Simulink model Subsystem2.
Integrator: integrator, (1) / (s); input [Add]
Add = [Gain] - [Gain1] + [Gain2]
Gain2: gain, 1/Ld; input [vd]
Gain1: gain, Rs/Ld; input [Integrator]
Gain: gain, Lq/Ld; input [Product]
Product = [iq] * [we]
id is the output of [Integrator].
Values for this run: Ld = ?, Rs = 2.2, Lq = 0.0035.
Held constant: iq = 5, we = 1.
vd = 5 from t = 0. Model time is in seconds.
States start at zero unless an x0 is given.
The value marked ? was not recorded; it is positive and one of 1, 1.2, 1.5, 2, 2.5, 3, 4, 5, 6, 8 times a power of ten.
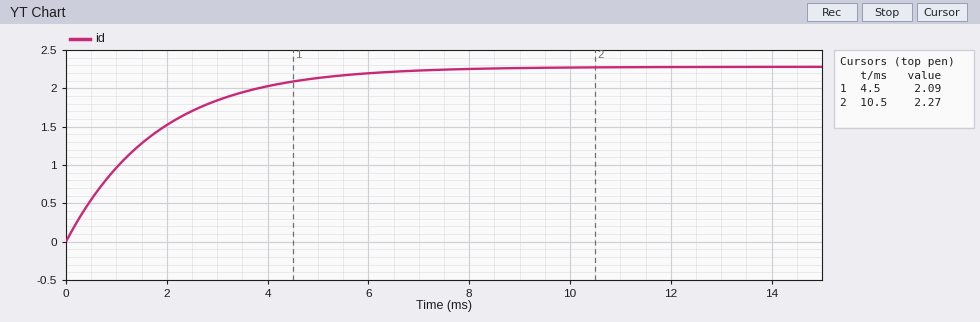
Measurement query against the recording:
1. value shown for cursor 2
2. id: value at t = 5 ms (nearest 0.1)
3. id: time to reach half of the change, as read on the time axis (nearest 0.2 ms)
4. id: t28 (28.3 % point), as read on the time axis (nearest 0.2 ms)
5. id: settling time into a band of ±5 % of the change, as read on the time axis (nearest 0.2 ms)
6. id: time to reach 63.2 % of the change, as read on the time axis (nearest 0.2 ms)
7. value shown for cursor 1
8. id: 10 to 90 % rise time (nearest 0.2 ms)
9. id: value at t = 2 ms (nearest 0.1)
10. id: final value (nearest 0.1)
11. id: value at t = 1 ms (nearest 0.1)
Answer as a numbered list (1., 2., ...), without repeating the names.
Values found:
1. 2.27
2. 2.1
3. 1.2 ms
4. 0.6 ms
5. 5.4 ms
6. 1.8 ms
7. 2.09
8. 4.0 ms
9. 1.5
10. 2.3
11. 1.0
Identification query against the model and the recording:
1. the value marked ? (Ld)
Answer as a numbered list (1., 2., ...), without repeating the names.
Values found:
1. 0.004
